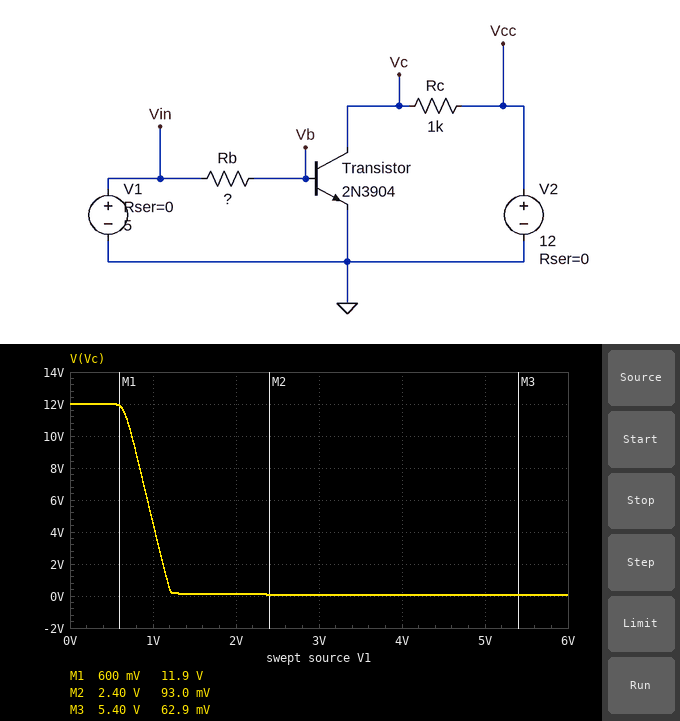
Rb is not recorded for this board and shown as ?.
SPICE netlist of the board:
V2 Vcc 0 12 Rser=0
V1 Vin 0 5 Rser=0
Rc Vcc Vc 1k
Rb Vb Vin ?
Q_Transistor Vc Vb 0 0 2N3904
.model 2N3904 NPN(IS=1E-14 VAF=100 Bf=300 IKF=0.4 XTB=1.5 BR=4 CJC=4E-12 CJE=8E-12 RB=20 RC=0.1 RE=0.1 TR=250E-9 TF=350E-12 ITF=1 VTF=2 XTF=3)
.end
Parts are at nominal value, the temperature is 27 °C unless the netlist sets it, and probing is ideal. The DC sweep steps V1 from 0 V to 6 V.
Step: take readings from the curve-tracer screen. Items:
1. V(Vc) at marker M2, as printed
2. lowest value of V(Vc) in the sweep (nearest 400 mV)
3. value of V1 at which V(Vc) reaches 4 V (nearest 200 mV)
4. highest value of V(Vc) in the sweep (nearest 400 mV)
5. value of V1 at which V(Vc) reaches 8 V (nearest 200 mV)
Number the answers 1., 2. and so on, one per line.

1. 93.0 mV
2. 0 V
3. 1.0 V
4. 12.0 V
5. 800 mV
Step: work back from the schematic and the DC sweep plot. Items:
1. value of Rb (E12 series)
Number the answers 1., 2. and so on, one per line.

1. 12 kΩ
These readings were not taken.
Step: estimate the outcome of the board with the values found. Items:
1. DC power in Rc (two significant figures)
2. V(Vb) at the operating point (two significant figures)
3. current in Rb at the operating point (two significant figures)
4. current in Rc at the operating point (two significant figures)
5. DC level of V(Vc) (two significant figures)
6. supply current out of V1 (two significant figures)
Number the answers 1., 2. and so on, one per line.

1. 140 mW
2. 730 mV
3. 360 µA
4. 12 mA
5. 65 mV
6. 360 µA
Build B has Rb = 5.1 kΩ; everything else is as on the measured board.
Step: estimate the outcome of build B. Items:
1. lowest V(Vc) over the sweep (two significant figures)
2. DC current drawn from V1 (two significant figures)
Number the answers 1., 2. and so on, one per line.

1. 41 mV
2. 830 µA
